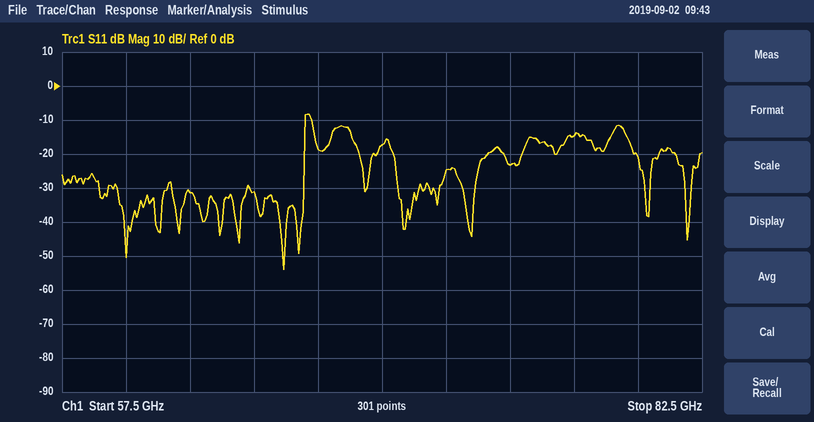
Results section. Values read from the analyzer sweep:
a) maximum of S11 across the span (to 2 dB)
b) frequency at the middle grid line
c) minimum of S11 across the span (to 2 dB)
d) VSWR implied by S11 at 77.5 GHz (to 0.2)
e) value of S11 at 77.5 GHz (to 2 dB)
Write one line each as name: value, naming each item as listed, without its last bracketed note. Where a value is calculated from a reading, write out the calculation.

maximum of S11 across the span: -8 dB
frequency at the middle grid line: 70 GHz
minimum of S11 across the span: -54 dB
VSWR implied by S11 at 77.5 GHz: |Γ| = 10^(-14/20) = 0.1995; VSWR = (1 + 0.1995)/(1 − 0.1995) ≈ 1.50, so 1.4 to the nearest 0.2
value of S11 at 77.5 GHz: -14 dB
